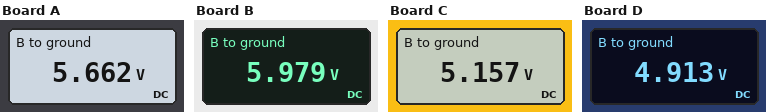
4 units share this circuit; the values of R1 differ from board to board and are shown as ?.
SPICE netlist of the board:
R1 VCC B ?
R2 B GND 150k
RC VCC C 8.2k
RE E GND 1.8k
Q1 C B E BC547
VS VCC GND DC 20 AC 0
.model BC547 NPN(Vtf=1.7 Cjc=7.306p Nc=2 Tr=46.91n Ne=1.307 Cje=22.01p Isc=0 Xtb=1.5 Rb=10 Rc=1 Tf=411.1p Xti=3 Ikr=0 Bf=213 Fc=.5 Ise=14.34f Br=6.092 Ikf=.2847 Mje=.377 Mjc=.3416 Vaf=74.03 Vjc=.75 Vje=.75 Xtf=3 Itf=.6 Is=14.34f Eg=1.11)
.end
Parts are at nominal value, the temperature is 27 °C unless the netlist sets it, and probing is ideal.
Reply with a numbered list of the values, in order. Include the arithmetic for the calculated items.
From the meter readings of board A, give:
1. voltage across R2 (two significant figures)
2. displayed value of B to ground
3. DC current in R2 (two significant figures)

1. 5.662 V = 5.7 V
2. 5.662 V
3. (5.662 V) / 150 kΩ = 38 µA
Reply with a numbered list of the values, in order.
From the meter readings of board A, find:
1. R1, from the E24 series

1. 15 kΩ
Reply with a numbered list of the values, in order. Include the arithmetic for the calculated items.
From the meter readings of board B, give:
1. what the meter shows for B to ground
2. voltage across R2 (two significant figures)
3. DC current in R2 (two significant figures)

1. 5.979 V
2. 5.979 V = 6.0 V
3. (5.979 V) / 150 kΩ = 40 µA
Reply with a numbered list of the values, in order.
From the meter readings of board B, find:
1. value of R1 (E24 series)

1. 12 kΩ
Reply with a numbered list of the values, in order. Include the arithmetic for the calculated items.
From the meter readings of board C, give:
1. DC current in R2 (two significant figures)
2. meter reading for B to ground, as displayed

1. (5.157 V) / 150 kΩ = 34 µA
2. 5.157 V
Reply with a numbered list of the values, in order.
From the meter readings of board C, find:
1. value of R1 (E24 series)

1. 24 kΩ
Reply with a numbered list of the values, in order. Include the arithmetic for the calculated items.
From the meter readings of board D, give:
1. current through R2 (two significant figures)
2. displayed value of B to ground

1. (4.913 V) / 150 kΩ = 33 µA
2. 4.913 V
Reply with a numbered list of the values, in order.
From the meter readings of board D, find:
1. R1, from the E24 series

1. 33 kΩ
